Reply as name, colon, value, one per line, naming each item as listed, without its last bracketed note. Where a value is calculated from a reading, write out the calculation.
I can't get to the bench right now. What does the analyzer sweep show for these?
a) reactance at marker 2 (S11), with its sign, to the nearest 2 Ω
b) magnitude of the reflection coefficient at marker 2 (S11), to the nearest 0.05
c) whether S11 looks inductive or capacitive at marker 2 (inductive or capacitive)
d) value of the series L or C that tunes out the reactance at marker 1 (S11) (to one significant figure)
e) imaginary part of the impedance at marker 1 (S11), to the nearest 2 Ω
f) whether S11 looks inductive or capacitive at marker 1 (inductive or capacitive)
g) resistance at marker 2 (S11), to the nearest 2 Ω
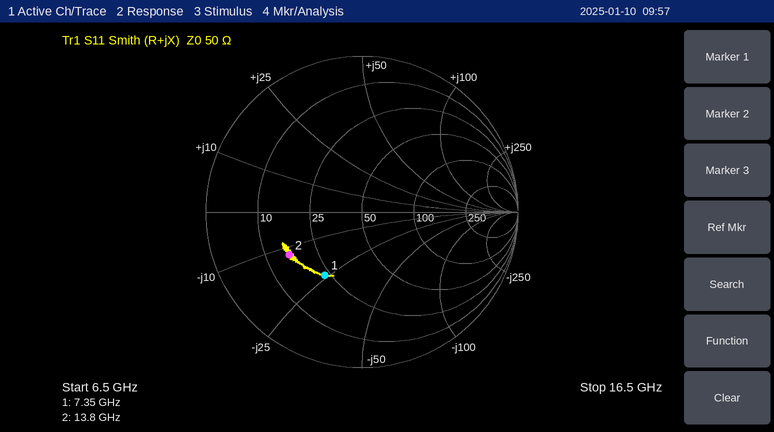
reactance at marker 2 (S11), with its sign, to the nearest 2 Ω: -12 Ω
magnitude of the reflection coefficient at marker 2 (S11), to the nearest 0.05: 0.55
whether S11 looks inductive or capacitive at marker 2: capacitive
value of the series L or C that tunes out the reactance at marker 1 (S11): L = 24 Ω/(2π × 7.35 GHz) ≈ 520 pH, so 500 pH to one significant figure
imaginary part of the impedance at marker 1 (S11), to the nearest 2 Ω: -24 Ω
whether S11 looks inductive or capacitive at marker 1: capacitive
resistance at marker 2 (S11), to the nearest 2 Ω: 16 Ω
